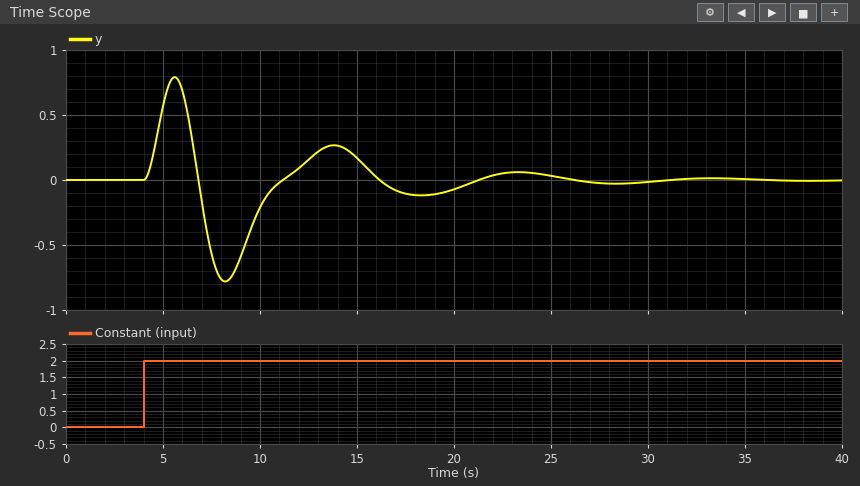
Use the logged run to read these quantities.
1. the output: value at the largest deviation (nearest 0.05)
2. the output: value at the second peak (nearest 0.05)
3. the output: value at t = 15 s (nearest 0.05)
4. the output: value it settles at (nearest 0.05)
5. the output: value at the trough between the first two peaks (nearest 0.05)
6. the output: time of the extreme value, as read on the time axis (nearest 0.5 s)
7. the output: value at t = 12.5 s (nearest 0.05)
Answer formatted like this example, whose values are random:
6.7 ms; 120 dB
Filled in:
0.80; 0.25; 0.15; 0.00; -0.80; 5.5 s; 0.15
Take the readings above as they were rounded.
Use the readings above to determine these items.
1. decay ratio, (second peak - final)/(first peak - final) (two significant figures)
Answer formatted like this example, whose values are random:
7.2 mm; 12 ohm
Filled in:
0.31
